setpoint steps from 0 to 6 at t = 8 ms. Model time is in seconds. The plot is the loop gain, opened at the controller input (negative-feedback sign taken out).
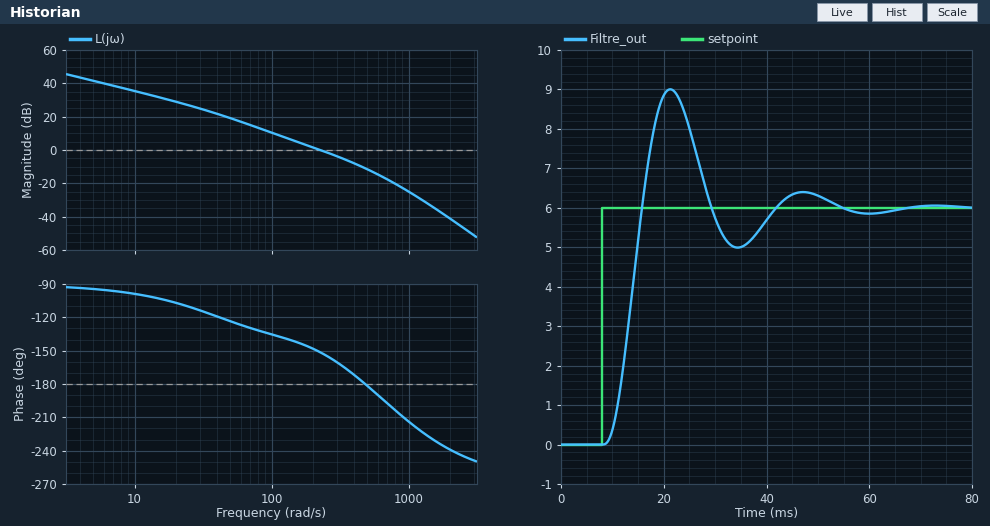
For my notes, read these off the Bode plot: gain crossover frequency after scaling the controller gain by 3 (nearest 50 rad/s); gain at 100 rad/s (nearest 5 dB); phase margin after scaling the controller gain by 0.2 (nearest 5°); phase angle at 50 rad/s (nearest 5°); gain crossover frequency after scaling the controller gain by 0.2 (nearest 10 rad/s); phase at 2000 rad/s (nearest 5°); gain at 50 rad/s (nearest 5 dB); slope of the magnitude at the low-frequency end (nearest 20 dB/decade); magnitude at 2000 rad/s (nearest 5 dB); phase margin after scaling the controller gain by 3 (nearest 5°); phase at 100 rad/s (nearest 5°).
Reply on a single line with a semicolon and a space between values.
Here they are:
450 rad/s; 10 dB; 50°; -125°; 80 rad/s; -240°; 20 dB; -20 dB/decade; -40 dB; 5°; -135°
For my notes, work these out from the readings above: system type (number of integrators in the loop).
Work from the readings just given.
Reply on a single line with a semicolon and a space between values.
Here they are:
1
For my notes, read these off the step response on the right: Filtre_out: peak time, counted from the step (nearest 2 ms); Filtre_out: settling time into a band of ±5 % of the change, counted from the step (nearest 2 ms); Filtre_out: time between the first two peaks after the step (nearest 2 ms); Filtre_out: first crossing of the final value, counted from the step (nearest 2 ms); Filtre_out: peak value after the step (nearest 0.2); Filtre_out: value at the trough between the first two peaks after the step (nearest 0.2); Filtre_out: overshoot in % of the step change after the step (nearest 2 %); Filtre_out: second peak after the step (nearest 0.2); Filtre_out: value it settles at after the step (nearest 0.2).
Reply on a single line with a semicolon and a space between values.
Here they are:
14 ms; 42 ms; 26 ms; 8 ms; 9.0; 5.0; 50 %; 6.4; 6.0
